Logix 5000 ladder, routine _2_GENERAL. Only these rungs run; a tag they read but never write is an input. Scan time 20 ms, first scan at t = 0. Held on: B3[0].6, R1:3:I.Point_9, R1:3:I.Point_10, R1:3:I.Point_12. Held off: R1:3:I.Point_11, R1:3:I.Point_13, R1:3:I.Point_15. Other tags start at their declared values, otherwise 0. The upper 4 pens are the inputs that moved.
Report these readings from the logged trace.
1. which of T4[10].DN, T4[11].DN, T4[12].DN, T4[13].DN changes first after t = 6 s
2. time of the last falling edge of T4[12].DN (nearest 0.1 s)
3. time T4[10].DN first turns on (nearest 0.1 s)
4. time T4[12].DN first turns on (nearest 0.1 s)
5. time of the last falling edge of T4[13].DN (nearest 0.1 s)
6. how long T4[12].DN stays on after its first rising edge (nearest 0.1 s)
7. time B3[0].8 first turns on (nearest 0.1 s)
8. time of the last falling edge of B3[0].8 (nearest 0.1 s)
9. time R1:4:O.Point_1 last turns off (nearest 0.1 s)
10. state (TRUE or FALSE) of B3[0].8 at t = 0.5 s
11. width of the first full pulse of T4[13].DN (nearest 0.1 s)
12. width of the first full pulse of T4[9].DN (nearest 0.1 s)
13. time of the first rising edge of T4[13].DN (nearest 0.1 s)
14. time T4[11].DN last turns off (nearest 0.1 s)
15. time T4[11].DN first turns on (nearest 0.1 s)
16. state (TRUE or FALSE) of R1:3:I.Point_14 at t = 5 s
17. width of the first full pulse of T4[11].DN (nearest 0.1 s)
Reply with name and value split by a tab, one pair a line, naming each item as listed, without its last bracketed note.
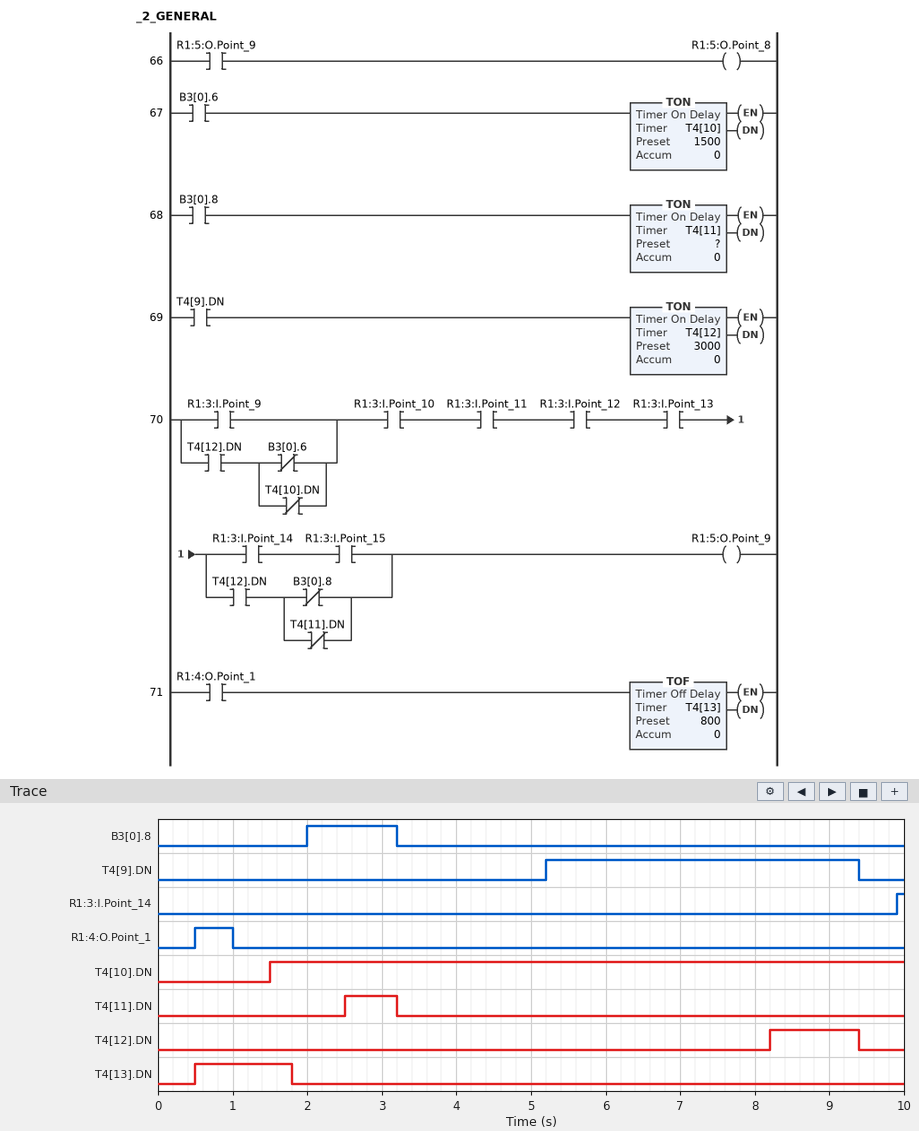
which of T4[10].DN, T4[11].DN, T4[12].DN, T4[13].DN changes first after t = 6 s	T4[12].DN
time of the last falling edge of T4[12].DN	9.4 s
time T4[10].DN first turns on	1.5 s
time T4[12].DN first turns on	8.2 s
time of the last falling edge of T4[13].DN	1.8 s
how long T4[12].DN stays on after its first rising edge	1.2 s
time B3[0].8 first turns on	2.0 s
time of the last falling edge of B3[0].8	3.2 s
time R1:4:O.Point_1 last turns off	1.0 s
state (TRUE or FALSE) of B3[0].8 at t = 0.5 s	FALSE
width of the first full pulse of T4[13].DN	1.3 s
width of the first full pulse of T4[9].DN	4.2 s
time of the first rising edge of T4[13].DN	0.5 s
time T4[11].DN last turns off	3.2 s
time T4[11].DN first turns on	2.5 s
state (TRUE or FALSE) of R1:3:I.Point_14 at t = 5 s	FALSE
width of the first full pulse of T4[11].DN	0.7 s
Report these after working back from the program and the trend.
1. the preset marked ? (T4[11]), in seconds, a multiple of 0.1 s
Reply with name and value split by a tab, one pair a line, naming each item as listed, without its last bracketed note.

the preset marked ? (T4[11]), in seconds, a multiple of 0.1 s	0.5 s
